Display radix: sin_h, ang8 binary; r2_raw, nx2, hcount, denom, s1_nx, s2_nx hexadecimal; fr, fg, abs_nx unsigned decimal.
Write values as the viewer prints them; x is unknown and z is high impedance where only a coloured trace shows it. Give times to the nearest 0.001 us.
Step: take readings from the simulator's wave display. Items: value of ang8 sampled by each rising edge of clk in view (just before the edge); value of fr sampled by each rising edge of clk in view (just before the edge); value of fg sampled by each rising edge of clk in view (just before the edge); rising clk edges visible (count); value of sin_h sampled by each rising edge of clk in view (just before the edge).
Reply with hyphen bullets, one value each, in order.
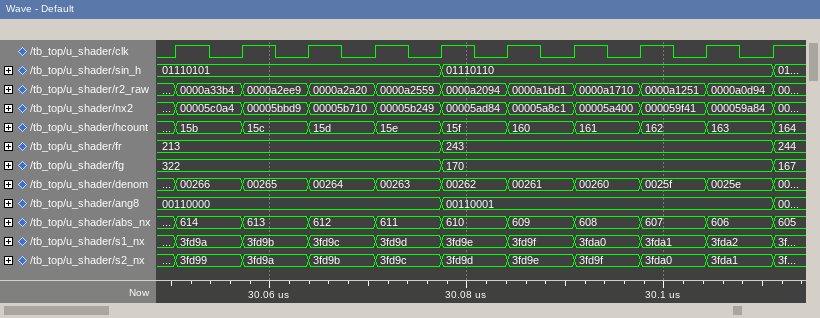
- 00110000, 00110000, 00110000, 00110000, 00110000, 00110001, 00110001, 00110001, 00110001, 00110001
- 213, 213, 213, 213, 213, 243, 243, 243, 243, 243
- 322, 322, 322, 322, 322, 170, 170, 170, 170, 170
- 10
- 01110101, 01110101, 01110101, 01110101, 01110101, 01110110, 01110110, 01110110, 01110110, 01110110
